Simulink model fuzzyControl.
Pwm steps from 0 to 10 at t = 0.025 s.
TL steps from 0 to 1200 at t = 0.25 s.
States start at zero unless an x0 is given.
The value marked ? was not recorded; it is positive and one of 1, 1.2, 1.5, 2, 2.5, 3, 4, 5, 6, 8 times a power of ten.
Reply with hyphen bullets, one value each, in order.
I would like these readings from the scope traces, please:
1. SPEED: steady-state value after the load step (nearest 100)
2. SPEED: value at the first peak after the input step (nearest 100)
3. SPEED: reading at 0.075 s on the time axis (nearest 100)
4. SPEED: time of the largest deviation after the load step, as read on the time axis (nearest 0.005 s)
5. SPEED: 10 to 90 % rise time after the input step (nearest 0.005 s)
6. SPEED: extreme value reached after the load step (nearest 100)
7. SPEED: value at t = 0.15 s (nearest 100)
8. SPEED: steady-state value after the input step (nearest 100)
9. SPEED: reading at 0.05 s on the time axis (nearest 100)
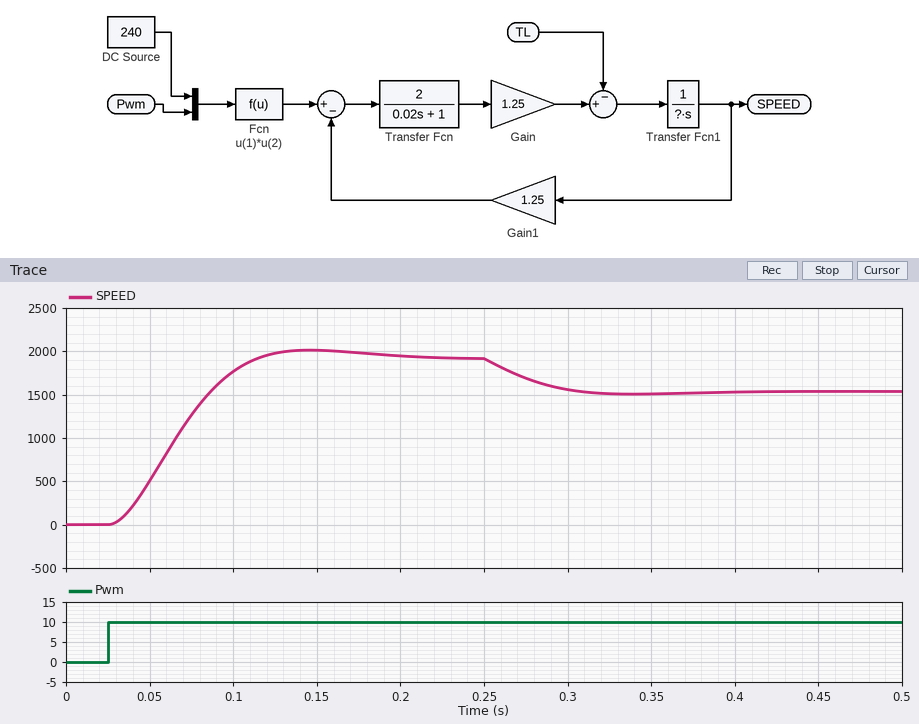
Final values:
- 1500
- 2000
- 1300
- 0.340 s
- 0.060 s
- 1500
- 2000
- 1900
- 500
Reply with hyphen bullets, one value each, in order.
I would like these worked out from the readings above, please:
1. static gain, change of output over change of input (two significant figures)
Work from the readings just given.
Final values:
- 190
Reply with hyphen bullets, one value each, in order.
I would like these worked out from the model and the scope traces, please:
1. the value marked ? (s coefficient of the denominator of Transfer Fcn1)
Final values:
- 0.12
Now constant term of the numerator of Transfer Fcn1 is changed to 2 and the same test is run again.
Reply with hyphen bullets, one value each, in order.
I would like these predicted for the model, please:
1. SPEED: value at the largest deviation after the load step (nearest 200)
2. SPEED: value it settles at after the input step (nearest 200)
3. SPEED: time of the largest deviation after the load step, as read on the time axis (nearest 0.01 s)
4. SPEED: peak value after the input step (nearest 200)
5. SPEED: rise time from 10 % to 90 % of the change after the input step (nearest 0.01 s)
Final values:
- 1400
- 2000
- 0.30 s
- 2200
- 0.03 s
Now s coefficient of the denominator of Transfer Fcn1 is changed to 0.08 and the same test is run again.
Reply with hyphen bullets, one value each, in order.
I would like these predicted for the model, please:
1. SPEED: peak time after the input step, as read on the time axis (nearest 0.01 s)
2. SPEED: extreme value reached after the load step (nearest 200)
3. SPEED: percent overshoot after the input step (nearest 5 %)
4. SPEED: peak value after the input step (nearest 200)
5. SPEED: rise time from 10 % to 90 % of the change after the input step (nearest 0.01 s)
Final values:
- 0.11 s
- 1400
- 10 %
- 2200
- 0.04 s
